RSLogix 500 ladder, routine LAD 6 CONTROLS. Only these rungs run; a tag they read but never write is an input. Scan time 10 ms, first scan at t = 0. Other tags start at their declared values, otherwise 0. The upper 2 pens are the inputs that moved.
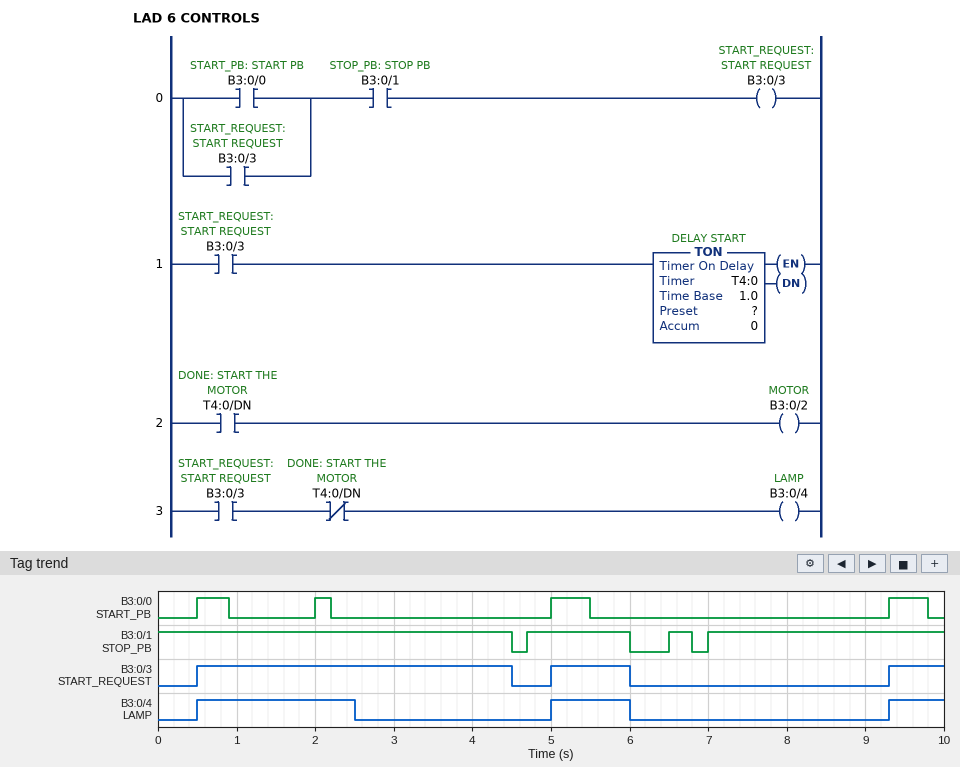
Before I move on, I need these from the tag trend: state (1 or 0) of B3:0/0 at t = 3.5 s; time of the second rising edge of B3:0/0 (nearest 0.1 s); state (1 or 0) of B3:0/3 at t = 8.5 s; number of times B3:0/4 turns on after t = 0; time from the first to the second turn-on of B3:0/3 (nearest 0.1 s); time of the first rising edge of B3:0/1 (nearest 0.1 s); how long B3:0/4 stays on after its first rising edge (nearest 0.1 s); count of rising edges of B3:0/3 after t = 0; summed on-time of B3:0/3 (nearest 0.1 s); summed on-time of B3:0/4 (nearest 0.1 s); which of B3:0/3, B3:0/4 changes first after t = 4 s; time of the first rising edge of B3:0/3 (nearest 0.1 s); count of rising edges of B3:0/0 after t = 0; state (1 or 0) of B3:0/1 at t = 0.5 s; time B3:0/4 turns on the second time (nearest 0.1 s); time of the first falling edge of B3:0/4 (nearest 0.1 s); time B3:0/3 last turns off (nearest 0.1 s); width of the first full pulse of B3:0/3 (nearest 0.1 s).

0
2.0 s
0
3
4.5 s
4.7 s
2.0 s
3
5.7 s
3.7 s
B3:0/3
0.5 s
4
1
5.0 s
2.5 s
6.0 s
4.0 s
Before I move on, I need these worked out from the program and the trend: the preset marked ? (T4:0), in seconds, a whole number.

2 s
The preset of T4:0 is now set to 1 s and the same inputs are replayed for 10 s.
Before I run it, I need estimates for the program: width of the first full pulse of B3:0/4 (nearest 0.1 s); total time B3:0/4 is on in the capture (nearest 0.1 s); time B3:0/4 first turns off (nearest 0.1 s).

1.0 s
2.7 s
1.5 s
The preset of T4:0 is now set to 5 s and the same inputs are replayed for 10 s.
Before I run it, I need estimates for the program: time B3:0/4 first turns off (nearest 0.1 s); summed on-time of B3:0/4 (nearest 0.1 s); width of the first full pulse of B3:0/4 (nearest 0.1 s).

4.5 s
5.7 s
4.0 s
